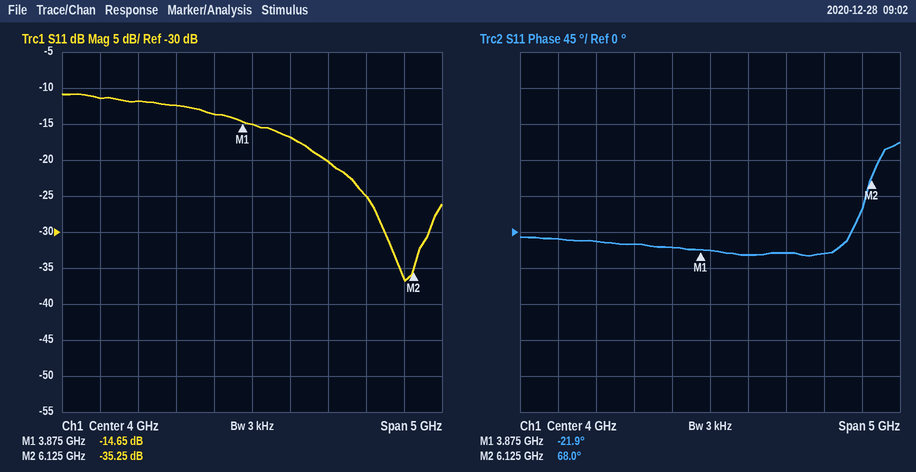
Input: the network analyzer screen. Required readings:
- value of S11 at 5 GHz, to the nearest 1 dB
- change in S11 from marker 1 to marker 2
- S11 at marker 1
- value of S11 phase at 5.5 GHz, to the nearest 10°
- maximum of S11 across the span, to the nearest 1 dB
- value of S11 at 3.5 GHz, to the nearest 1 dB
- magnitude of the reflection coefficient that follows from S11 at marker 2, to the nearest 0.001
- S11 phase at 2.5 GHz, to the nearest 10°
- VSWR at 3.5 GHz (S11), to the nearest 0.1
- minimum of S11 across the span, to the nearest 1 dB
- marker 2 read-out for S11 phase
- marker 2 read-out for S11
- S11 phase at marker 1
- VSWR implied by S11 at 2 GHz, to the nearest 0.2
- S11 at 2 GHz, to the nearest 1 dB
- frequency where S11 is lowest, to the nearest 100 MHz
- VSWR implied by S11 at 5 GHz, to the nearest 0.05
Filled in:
-20 dB
-20.60 dB
-14.65 dB
-30°
-11 dB
-14 dB
0.017
-10°
1.5
-37 dB
68.0°
-35.25 dB
-21.9°
1.8
-11 dB
6.0 GHz
1.20
